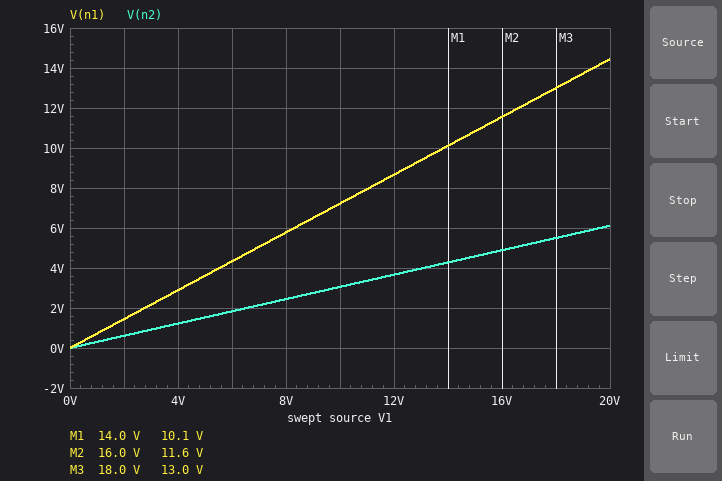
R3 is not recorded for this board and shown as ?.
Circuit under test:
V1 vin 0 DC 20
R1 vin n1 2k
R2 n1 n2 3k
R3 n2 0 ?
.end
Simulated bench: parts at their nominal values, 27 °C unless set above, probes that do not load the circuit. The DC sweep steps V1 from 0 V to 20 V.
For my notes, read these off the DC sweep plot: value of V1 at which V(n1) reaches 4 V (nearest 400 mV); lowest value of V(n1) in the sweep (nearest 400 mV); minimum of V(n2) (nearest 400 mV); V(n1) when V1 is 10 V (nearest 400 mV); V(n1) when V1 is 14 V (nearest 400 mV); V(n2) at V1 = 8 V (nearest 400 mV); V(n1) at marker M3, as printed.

5.6 V
0 V
0 V
7.2 V
10.0 V
2.4 V
13.0 V
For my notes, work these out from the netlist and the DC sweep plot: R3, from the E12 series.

2.2 kΩ
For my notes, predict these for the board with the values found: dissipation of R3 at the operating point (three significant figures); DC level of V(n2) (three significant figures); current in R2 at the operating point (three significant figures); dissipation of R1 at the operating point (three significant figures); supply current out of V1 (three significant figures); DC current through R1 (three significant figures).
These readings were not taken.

17.0 mW
6.11 V
2.78 mA
15.4 mW
2.78 mA
2.78 mA
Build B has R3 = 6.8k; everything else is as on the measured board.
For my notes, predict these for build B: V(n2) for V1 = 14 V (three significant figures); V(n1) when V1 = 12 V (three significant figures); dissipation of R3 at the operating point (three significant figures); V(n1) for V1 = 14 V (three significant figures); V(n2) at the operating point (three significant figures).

8.07 V
9.97 V
19.5 mW
11.6 V
11.5 V
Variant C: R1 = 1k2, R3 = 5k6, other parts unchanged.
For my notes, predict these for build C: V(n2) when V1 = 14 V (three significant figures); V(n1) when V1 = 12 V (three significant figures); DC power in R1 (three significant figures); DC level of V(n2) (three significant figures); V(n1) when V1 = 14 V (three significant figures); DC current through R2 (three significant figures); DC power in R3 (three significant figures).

8.00 V
10.5 V
5.00 mW
11.4 V
12.3 V
2.04 mA
23.3 mW
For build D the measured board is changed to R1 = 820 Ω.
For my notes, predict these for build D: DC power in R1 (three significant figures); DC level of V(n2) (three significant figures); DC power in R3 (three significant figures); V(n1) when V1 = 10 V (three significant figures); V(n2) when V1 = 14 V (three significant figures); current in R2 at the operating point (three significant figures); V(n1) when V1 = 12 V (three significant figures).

9.05 mW
7.31 V
24.3 mW
8.64 V
5.12 V
3.32 mA
10.4 V
